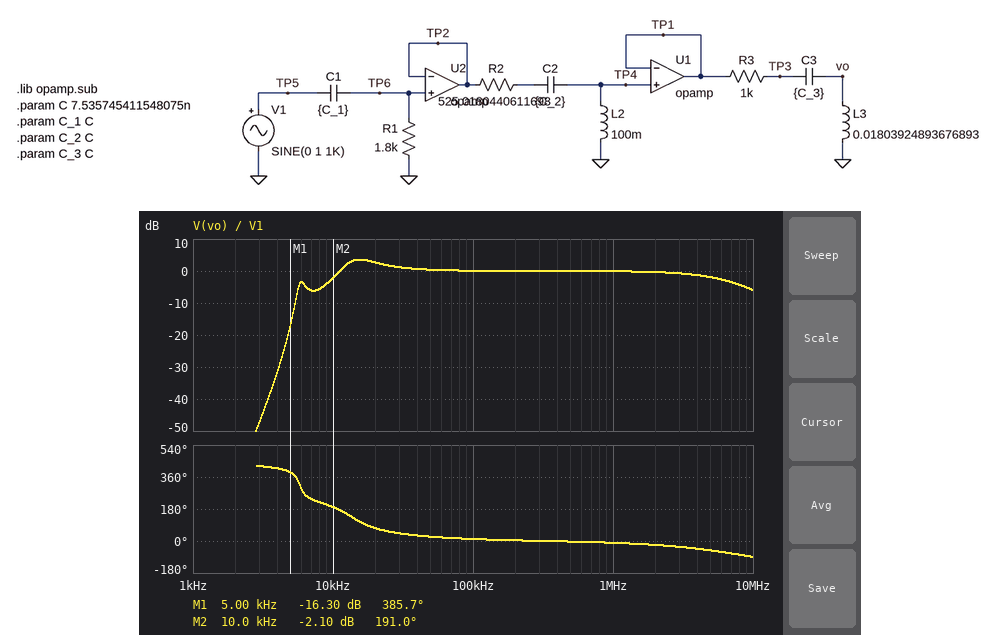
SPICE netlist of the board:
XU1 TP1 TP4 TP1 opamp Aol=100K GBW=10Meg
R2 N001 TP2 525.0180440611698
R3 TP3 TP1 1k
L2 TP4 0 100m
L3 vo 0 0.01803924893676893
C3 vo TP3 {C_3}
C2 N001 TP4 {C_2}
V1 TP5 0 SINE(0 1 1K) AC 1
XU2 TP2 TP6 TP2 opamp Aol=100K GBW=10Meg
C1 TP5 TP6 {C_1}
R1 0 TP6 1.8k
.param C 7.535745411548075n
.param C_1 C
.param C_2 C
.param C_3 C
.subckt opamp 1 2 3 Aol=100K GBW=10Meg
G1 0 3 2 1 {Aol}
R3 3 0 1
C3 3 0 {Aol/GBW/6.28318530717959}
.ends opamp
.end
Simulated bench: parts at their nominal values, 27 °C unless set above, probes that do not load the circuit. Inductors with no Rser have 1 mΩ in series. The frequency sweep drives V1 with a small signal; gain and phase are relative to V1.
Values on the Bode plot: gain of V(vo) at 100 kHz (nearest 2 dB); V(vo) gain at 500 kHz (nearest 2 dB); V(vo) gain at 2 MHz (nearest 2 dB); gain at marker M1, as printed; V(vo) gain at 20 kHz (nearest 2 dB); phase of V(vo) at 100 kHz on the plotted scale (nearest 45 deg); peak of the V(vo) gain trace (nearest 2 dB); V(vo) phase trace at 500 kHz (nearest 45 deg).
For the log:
0 dB
0 dB
0 dB
-16.30 dB
2 dB
0 deg
4 dB
0 deg
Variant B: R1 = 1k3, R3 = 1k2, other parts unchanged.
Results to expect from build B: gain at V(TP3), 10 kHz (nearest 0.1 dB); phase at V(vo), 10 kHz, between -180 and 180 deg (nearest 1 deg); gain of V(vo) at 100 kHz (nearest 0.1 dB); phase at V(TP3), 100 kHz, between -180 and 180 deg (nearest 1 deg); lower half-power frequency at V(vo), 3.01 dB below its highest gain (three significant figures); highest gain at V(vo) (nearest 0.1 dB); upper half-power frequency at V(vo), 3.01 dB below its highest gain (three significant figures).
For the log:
-6.1 dB
-165 deg
0 dB
15 deg
11.8 kHz
1.1 dB
4.90 MHz
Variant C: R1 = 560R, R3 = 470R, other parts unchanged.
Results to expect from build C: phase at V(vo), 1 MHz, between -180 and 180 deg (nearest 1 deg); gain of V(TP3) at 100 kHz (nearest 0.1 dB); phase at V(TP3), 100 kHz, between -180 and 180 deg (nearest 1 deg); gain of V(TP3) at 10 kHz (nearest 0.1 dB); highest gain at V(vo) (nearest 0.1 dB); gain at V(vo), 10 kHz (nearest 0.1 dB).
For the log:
-9 deg
-0.6 dB
22 deg
-9.2 dB
2.9 dB
-8.0 dB
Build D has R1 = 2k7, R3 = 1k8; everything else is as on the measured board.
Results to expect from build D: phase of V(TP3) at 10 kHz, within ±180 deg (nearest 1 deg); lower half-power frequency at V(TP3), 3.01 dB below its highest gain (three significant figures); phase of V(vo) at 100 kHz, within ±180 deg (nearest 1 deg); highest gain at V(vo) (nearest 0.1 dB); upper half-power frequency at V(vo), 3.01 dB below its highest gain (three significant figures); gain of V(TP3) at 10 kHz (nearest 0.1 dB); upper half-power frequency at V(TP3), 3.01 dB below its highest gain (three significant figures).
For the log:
-16 deg
5.46 kHz
13 deg
0.6 dB
5.70 MHz
-5.0 dB
6.32 kHz
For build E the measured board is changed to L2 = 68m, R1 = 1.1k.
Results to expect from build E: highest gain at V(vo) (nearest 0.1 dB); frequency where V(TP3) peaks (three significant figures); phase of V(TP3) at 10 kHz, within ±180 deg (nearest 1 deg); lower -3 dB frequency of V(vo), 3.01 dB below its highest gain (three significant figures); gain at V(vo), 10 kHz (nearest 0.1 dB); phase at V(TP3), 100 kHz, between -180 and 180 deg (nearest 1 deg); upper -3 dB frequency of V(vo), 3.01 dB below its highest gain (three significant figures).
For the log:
2.2 dB
7.12 kHz
30 deg
11.4 kHz
-2.9 dB
16 deg
3.15 MHz
